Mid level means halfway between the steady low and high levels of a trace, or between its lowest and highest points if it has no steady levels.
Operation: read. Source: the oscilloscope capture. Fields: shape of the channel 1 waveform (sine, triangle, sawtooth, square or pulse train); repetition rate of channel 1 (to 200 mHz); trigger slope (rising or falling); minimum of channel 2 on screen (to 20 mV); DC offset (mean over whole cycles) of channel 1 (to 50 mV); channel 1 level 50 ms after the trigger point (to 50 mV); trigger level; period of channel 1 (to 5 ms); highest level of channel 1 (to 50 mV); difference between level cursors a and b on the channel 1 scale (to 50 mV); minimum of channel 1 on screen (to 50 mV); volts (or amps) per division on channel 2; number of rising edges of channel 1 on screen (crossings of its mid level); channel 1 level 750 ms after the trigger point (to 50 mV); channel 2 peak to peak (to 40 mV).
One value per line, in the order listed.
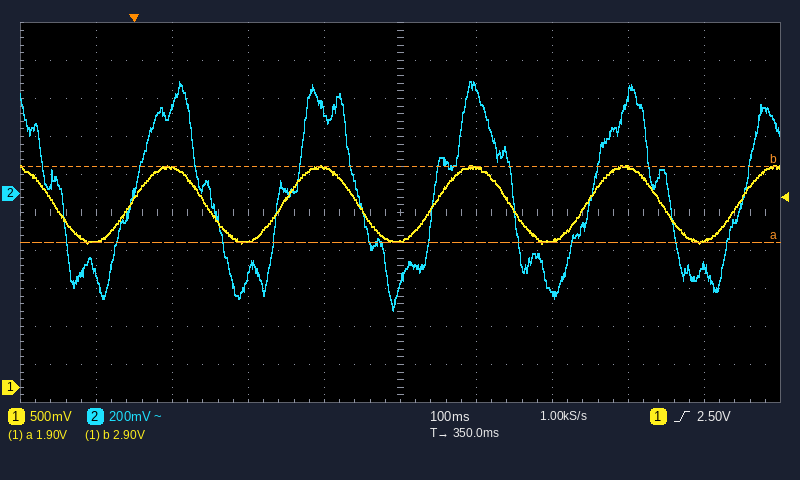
sine
5.0 Hz
rising
-620 mV
2.40 V
2.90 V
2.50 V
200 ms
2.90 V
1.00 V
1.90 V
200 mV
5
1.95 V
1.20 V
